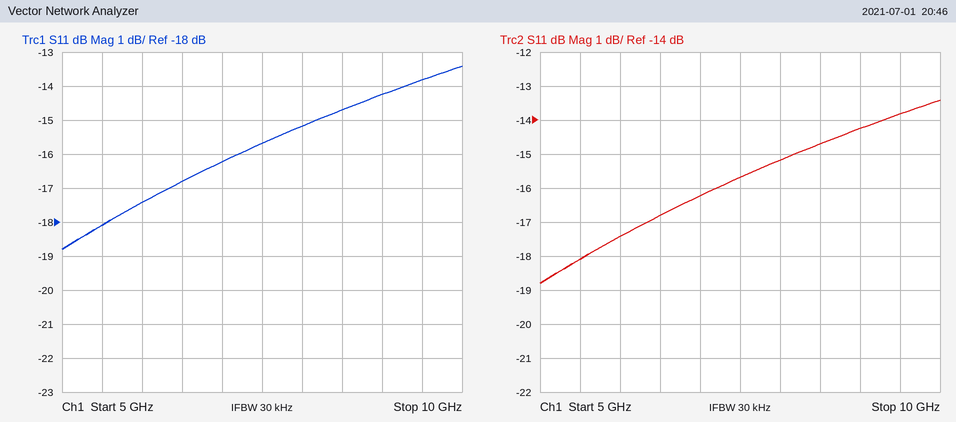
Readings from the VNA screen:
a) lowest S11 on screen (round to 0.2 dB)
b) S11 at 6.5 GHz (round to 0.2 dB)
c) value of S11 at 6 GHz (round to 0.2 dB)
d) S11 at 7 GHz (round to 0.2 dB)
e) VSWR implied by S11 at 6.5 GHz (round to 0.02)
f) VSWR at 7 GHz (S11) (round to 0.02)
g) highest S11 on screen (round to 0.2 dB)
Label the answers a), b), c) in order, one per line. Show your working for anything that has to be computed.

a) -18.8 dB
b) -16.8 dB
c) -17.4 dB
d) -16.2 dB
e) |Γ| = 10^(-16.8/20) = 0.1445; VSWR = (1 + 0.1445)/(1 − 0.1445) ≈ 1.34
f) |Γ| = 10^(-16.2/20) = 0.1549; VSWR = (1 + 0.1549)/(1 − 0.1549) ≈ 1.37, so 1.36 to the nearest 0.02
g) -13.4 dB
